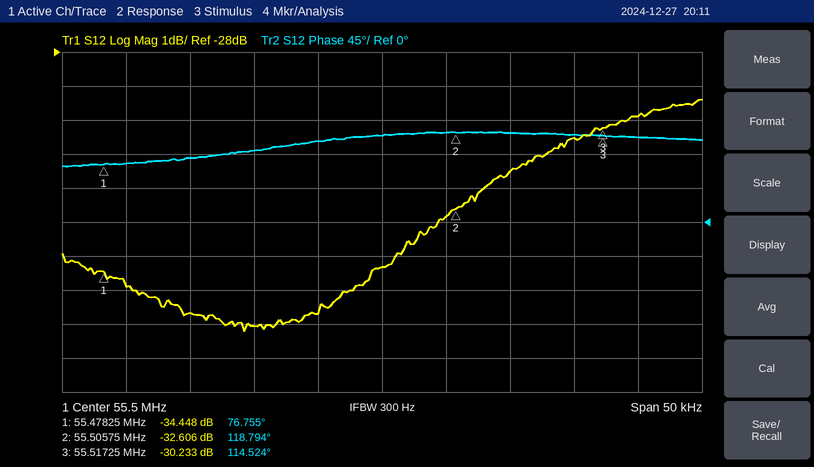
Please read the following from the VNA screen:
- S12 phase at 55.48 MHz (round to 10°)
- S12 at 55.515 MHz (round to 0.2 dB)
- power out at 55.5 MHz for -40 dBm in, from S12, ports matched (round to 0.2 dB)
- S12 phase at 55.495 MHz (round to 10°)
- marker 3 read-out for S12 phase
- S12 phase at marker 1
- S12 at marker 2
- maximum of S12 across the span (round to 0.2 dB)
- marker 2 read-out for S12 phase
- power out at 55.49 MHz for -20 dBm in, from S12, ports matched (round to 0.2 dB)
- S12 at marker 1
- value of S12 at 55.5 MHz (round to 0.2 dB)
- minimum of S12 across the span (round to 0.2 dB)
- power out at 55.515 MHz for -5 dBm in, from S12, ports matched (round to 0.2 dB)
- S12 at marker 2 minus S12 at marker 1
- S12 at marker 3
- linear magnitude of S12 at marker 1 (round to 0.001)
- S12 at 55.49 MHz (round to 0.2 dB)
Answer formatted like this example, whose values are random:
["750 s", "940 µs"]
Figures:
["80°", "-30.6 dB", "-74.4 dBm", "110°", "114.524°", "76.755°", "-32.606 dB", "-29.4 dB", "118.794°", "-56.0 dBm", "-34.448 dB", "-34.4 dB", "-36.2 dB", "-35.6 dBm", "1.842 dB", "-30.233 dB", "0.019", "-36.0 dB"]
